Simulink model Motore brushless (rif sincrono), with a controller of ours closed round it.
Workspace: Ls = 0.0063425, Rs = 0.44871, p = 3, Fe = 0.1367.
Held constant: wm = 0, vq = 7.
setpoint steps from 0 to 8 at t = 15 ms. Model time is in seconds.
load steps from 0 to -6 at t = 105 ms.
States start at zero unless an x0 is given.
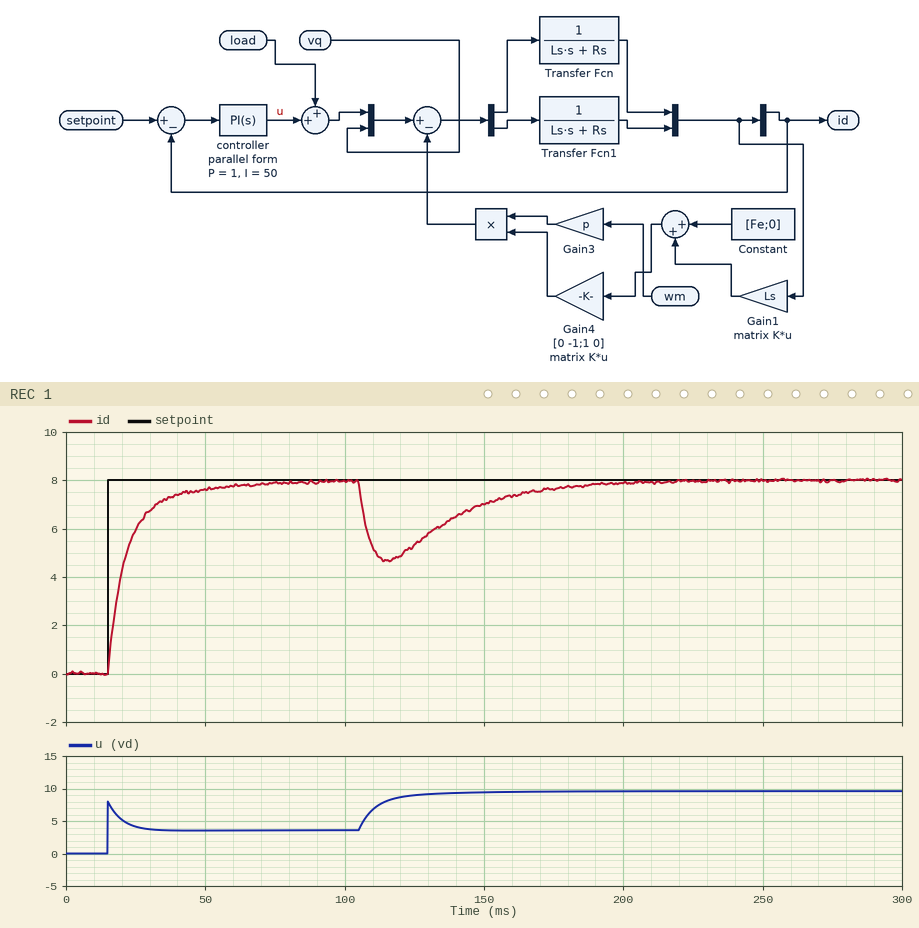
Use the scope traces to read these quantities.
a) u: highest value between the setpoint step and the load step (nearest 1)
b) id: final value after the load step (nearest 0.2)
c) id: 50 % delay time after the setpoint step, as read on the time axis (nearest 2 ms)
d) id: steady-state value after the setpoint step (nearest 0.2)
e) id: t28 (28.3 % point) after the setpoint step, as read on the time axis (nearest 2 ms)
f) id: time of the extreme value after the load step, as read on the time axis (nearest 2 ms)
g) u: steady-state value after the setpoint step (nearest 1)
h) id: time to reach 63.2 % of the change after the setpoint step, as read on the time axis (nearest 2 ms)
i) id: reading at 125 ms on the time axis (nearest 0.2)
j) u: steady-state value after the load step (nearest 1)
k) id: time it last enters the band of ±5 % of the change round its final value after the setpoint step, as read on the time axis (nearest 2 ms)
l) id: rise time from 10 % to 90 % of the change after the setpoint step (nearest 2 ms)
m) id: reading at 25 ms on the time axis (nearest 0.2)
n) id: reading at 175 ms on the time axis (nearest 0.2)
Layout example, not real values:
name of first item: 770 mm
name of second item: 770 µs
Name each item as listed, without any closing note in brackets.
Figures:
u: highest value between the setpoint step and the load step: 8
id: final value after the load step: 8.0
id: 50 % delay time after the setpoint step, as read on the time axis: 20 ms
id: steady-state value after the setpoint step: 8.0
id: t28 (28.3 % point) after the setpoint step, as read on the time axis: 18 ms
id: time of the extreme value after the load step, as read on the time axis: 116 ms
u: steady-state value after the setpoint step: 4
id: time to reach 63.2 % of the change after the setpoint step, as read on the time axis: 22 ms
id: reading at 125 ms on the time axis: 5.4
u: steady-state value after the load step: 10
id: time it last enters the band of ±5 % of the change round its final value after the setpoint step, as read on the time axis: 48 ms
id: rise time from 10 % to 90 % of the change after the setpoint step: 20 ms
id: reading at 25 ms on the time axis: 6.0
id: reading at 175 ms on the time axis: 7.6
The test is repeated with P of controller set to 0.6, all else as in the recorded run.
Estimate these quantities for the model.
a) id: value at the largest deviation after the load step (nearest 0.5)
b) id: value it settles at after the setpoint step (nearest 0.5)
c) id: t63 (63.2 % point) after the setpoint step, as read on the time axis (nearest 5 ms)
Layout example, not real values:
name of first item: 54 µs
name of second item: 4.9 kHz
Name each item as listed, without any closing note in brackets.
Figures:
id: value at the largest deviation after the load step: 4.0
id: value it settles at after the setpoint step: 8.0
id: t63 (63.2 % point) after the setpoint step, as read on the time axis: 25 ms
